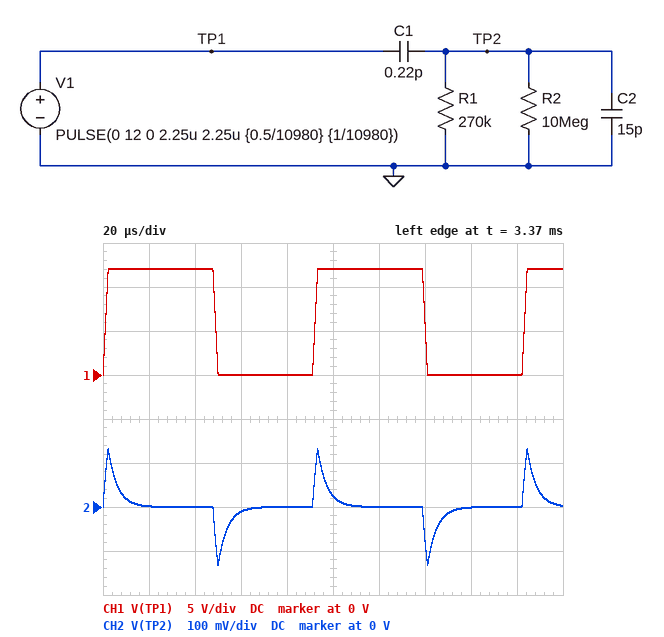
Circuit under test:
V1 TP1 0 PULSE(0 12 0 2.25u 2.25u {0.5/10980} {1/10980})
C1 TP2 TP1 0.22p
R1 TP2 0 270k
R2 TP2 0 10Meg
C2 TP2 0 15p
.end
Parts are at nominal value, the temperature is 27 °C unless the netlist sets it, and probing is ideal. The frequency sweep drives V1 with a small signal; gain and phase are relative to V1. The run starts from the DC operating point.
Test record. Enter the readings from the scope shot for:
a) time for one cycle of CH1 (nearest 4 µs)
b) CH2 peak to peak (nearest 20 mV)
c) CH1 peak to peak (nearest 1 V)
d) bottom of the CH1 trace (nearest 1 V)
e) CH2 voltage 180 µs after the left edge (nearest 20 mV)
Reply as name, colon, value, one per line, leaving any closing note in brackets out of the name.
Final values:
time for one cycle of CH1: 92 µs
CH2 peak to peak: 260 mV
CH1 peak to peak: 12 V
bottom of the CH1 trace: 0 V
CH2 voltage 180 µs after the left edge: 0 V
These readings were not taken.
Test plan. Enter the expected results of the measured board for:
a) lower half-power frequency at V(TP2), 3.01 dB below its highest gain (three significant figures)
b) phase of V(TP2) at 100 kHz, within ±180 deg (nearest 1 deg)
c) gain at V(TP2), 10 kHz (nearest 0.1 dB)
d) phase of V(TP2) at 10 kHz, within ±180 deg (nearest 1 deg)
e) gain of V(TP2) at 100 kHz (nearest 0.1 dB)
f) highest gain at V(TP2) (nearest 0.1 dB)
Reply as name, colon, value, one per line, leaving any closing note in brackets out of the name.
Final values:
lower half-power frequency at V(TP2), 3.01 dB below its highest gain: 39.8 kHz
phase of V(TP2) at 100 kHz, within ±180 deg: 22 deg
gain at V(TP2), 10 kHz: -49.1 dB
phase of V(TP2) at 10 kHz, within ±180 deg: 76 deg
gain of V(TP2) at 100 kHz: -37.4 dB
highest gain at V(TP2): -36.8 dB
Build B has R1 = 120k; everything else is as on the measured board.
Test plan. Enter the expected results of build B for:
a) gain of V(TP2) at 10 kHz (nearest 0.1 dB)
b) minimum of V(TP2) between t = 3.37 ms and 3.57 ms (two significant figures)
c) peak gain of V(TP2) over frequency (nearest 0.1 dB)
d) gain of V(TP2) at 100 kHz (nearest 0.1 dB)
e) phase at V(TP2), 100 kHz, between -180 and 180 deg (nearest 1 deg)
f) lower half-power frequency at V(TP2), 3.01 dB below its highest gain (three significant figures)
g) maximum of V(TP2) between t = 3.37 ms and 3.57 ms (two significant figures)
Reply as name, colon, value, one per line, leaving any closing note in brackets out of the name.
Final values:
gain of V(TP2) at 10 kHz: -55.8 dB
minimum of V(TP2) between t = 3.37 ms and 3.57 ms: -99 mV
peak gain of V(TP2) over frequency: -36.8 dB
gain of V(TP2) at 100 kHz: -39.3 dB
phase at V(TP2), 100 kHz, between -180 and 180 deg: 41 deg
lower half-power frequency at V(TP2), 3.01 dB below its highest gain: 88.2 kHz
maximum of V(TP2) between t = 3.37 ms and 3.57 ms: 99 mV
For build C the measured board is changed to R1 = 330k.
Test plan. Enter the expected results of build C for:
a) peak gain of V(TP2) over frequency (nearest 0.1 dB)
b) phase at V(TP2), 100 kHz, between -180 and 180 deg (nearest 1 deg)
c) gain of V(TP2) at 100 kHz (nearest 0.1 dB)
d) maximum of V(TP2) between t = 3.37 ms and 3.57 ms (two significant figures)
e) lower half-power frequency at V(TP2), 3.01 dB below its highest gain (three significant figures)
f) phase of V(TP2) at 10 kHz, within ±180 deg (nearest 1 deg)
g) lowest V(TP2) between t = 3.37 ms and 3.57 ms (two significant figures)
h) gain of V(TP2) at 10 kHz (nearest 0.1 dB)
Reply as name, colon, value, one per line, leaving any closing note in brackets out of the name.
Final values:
peak gain of V(TP2) over frequency: -36.8 dB
phase at V(TP2), 100 kHz, between -180 and 180 deg: 18 deg
gain of V(TP2) at 100 kHz: -37.2 dB
maximum of V(TP2) between t = 3.37 ms and 3.57 ms: 140 mV
lower half-power frequency at V(TP2), 3.01 dB below its highest gain: 32.7 kHz
phase of V(TP2) at 10 kHz, within ±180 deg: 73 deg
lowest V(TP2) between t = 3.37 ms and 3.57 ms: -140 mV
gain of V(TP2) at 10 kHz: -47.5 dB
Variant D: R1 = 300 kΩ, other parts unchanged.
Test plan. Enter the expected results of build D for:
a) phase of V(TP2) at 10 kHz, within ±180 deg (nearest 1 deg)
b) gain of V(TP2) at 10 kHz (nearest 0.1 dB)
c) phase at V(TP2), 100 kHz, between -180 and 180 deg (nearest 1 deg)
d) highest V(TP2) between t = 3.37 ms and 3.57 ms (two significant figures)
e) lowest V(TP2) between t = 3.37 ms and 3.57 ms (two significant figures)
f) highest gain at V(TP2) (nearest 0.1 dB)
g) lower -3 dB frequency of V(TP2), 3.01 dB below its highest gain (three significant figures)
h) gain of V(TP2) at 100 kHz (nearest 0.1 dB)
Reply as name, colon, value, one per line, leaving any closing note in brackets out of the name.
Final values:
phase of V(TP2) at 10 kHz, within ±180 deg: 74 deg
gain of V(TP2) at 10 kHz: -48.2 dB
phase at V(TP2), 100 kHz, between -180 and 180 deg: 20 deg
highest V(TP2) between t = 3.37 ms and 3.57 ms: 140 mV
lowest V(TP2) between t = 3.37 ms and 3.57 ms: -140 mV
highest gain at V(TP2): -36.8 dB
lower -3 dB frequency of V(TP2), 3.01 dB below its highest gain: 35.9 kHz
gain of V(TP2) at 100 kHz: -37.3 dB
